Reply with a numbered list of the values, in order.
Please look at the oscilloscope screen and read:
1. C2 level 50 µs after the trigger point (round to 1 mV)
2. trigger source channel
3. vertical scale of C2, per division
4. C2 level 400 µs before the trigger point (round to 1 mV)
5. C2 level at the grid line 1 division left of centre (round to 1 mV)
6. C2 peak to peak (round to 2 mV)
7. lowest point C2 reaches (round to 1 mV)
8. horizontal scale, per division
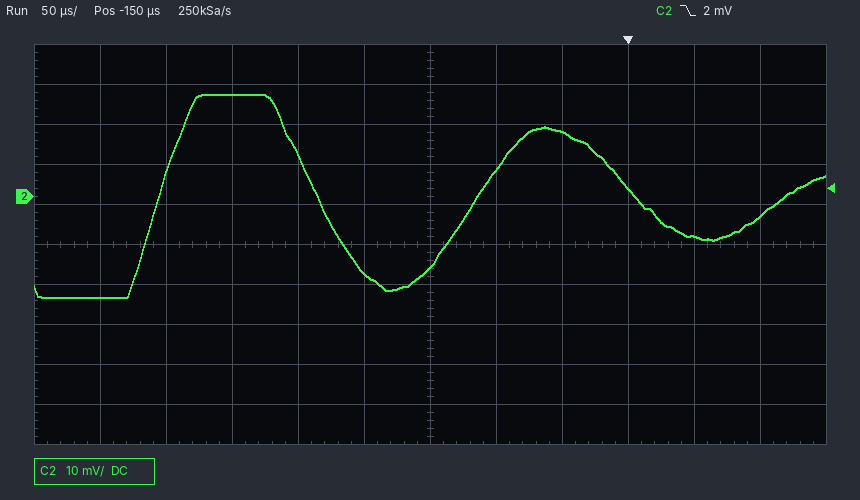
1. -10 mV
2. C2
3. 10 mV
4. -25 mV
5. -19 mV
6. 50 mV
7. -25 mV
8. 50 µs
